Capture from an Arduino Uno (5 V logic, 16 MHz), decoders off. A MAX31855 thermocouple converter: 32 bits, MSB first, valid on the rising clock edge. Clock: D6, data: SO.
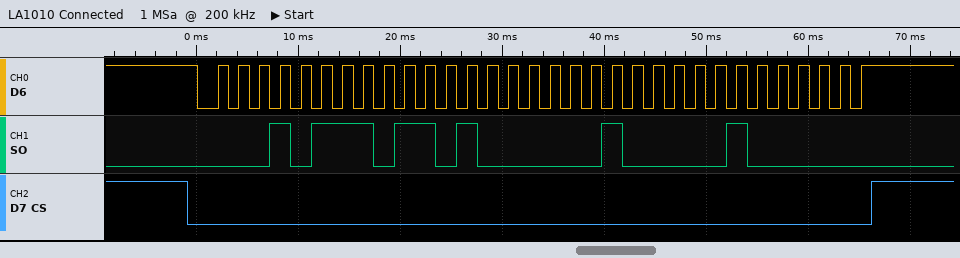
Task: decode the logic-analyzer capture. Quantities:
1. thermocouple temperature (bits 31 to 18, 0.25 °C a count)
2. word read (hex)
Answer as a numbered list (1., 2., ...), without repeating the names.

1. 374.50 °C
2. 0x17681040
